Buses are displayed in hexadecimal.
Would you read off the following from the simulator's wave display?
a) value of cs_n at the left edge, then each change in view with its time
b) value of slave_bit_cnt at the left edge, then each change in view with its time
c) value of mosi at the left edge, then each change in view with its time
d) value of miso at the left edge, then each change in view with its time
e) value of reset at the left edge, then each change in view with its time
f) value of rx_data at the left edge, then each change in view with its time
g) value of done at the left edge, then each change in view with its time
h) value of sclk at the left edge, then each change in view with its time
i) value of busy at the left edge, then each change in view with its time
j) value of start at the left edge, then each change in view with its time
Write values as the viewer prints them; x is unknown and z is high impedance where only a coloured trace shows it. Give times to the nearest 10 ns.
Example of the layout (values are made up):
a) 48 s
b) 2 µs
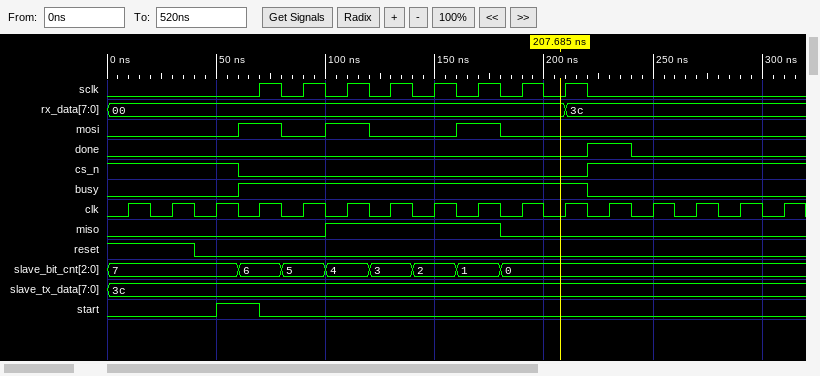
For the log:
a) 1, 0 at 60 ns, 1 at 220 ns
b) 7, 6 at 60 ns, 5 at 80 ns, 4 at 100 ns, 3 at 120 ns, 2 at 140 ns, 1 at 160 ns, 0 at 180 ns
c) 0, 1 at 60 ns, 0 at 80 ns, 1 at 100 ns, 0 at 120 ns, 1 at 160 ns, 0 at 180 ns
d) 0, 1 at 100 ns, 0 at 180 ns
e) 1, 0 at 40 ns
f) 00, 3c at 210 ns
g) 0, 1 at 220 ns, 0 at 240 ns
h) 0, 1 at 70 ns, 0 at 80 ns, 1 at 90 ns, 0 at 100 ns, 1 at 110 ns, 0 at 120 ns, 1 at 130 ns, 0 at 140 ns, 1 at 150 ns, 0 at 160 ns, 1 at 170 ns, 0 at 180 ns, 1 at 190 ns, 0 at 200 ns, 1 at 210 ns, 0 at 220 ns
i) 0, 1 at 60 ns, 0 at 220 ns
j) 0, 1 at 50 ns, 0 at 70 ns
